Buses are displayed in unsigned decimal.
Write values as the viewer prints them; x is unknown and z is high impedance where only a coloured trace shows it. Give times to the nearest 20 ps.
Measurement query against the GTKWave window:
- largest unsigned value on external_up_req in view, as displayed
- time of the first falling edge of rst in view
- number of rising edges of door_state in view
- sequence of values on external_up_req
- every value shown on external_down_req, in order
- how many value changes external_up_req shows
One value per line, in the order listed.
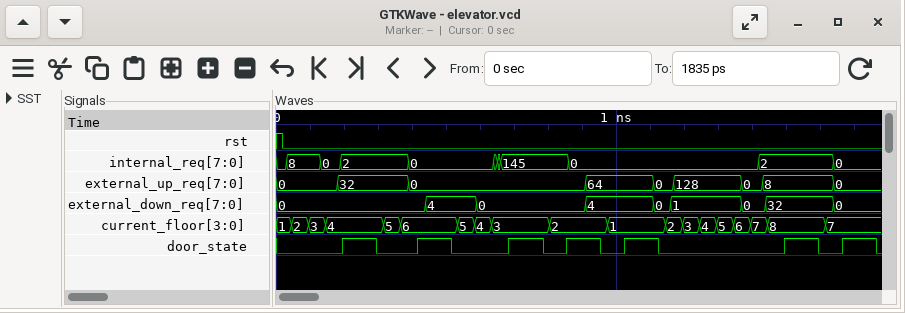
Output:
128
20 ps
7
0, 32, 0, 64, 0, 128, 0, 8, 0
0, 4, 0, 4, 0, 1, 0, 32, 0
8
